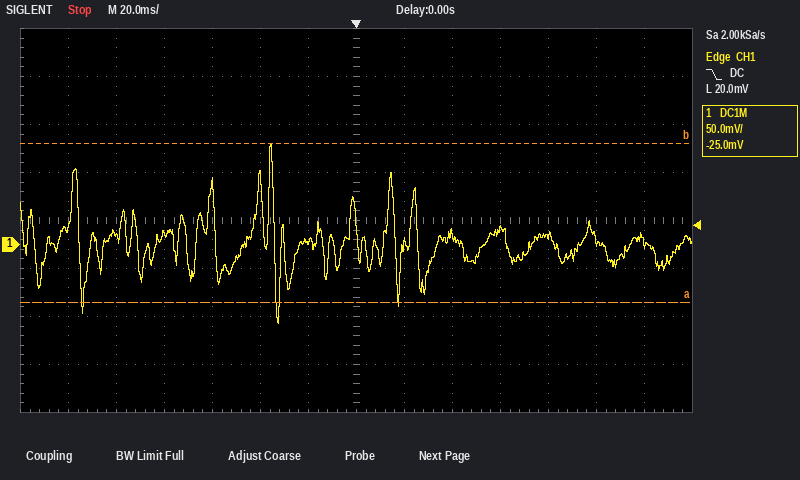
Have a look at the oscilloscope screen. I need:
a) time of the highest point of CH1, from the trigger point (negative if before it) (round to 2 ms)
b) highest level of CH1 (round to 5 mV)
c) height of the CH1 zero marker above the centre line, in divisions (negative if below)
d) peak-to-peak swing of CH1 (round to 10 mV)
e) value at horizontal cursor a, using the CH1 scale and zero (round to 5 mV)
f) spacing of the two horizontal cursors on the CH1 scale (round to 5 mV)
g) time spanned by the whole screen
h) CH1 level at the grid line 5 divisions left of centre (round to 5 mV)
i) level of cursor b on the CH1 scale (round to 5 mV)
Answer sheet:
-36 ms
105 mV
-0.5 div
190 mV
-60 mV
165 mV
280 ms
10 mV
105 mV
